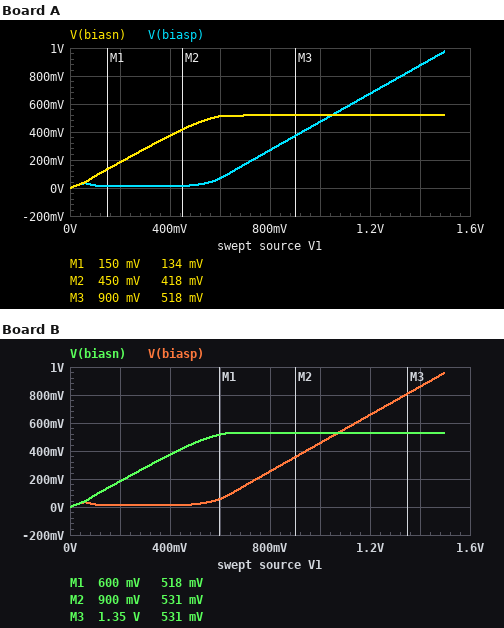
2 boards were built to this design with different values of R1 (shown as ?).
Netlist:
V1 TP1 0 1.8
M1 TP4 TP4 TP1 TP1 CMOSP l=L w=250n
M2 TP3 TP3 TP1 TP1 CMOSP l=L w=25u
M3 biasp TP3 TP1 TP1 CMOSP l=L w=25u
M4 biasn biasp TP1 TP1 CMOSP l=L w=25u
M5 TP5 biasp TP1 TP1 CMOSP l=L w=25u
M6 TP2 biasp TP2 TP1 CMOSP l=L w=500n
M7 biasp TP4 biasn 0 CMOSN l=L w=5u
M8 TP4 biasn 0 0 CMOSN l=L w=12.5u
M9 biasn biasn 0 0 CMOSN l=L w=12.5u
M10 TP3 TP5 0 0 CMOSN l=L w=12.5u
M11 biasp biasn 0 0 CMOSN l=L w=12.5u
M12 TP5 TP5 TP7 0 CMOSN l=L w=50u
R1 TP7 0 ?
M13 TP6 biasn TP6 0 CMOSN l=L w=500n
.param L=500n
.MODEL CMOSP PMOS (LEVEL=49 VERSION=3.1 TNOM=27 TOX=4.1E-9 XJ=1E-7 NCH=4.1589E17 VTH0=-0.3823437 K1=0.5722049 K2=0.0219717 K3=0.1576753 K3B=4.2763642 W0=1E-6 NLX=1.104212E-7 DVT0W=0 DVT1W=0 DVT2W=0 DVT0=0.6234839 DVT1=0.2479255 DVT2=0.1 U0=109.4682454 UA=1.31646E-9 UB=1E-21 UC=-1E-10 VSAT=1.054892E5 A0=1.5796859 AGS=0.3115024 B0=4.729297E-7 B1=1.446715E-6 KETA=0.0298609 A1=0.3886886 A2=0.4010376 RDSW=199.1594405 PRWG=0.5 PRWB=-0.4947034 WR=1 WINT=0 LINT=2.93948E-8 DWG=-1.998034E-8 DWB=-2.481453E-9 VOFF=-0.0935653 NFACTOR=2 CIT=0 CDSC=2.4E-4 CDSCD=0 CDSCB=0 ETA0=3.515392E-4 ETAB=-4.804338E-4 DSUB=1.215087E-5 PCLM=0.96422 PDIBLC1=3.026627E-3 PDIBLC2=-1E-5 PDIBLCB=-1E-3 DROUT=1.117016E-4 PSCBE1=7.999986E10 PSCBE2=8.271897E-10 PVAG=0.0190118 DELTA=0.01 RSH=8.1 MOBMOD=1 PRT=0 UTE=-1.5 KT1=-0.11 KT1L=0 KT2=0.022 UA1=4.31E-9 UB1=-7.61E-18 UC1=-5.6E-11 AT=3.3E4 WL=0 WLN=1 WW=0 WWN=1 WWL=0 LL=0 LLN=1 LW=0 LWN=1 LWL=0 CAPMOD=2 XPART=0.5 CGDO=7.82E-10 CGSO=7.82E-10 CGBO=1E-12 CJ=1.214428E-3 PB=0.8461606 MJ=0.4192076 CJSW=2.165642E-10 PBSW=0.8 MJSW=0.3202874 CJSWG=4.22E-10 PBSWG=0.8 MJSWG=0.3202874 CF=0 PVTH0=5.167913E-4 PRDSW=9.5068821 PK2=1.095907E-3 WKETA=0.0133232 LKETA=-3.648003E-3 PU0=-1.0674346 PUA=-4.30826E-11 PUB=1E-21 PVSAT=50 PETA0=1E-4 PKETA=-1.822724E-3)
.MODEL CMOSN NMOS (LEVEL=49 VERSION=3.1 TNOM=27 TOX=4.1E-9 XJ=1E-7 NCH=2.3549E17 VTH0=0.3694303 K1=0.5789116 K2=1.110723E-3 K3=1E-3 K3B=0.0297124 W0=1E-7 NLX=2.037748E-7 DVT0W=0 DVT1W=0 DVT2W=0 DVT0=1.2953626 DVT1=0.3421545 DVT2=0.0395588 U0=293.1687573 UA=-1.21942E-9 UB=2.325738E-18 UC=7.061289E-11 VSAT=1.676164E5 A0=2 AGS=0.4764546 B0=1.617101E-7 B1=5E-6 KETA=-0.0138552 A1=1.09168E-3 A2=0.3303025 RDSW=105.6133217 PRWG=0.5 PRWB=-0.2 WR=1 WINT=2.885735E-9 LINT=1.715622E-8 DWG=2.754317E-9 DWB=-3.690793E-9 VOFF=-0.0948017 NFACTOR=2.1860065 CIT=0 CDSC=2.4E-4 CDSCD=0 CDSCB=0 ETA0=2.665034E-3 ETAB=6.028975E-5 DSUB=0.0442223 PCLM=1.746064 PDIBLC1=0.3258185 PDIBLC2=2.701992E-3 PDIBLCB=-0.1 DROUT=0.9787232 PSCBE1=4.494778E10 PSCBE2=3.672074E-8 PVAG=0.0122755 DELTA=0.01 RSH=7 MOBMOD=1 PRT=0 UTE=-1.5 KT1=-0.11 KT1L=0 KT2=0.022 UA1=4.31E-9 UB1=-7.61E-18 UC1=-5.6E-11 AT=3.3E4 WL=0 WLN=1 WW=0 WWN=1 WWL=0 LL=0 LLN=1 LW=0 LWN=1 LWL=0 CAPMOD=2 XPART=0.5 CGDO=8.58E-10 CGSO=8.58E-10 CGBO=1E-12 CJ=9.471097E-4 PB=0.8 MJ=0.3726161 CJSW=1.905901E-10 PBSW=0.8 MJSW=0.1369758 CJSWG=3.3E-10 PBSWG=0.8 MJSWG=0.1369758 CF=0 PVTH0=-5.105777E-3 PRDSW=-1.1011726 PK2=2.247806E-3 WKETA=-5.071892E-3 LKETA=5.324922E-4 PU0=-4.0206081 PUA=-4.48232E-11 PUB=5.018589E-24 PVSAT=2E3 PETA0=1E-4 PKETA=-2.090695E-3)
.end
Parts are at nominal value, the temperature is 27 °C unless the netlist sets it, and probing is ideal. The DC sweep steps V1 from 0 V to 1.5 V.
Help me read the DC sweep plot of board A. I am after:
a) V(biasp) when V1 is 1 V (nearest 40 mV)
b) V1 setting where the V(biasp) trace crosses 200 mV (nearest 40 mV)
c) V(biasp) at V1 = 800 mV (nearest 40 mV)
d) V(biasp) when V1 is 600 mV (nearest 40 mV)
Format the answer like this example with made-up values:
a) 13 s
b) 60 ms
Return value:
a) 480 mV
b) 720 mV
c) 280 mV
d) 80 mV
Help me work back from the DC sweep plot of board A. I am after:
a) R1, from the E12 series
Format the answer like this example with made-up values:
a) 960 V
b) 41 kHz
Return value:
a) 2.7 kΩ
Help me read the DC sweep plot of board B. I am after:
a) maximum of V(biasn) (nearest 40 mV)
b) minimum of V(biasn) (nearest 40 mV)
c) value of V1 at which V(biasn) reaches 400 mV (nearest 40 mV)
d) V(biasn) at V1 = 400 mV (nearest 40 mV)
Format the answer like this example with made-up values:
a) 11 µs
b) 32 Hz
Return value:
a) 520 mV
b) 0 V
c) 440 mV
d) 360 mV
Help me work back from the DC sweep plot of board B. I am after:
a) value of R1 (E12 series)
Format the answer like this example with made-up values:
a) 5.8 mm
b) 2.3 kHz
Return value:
a) 2.2 kΩ
